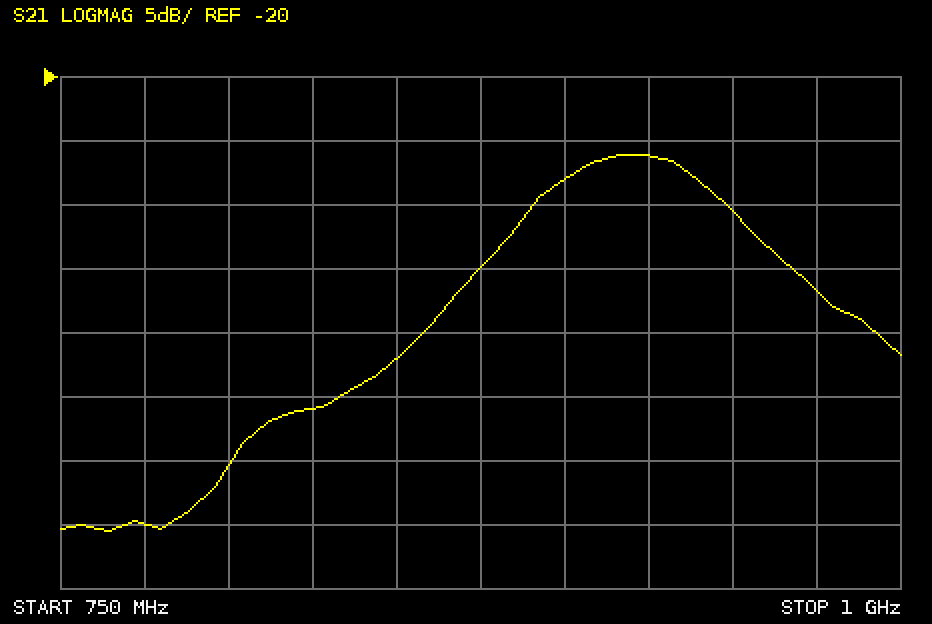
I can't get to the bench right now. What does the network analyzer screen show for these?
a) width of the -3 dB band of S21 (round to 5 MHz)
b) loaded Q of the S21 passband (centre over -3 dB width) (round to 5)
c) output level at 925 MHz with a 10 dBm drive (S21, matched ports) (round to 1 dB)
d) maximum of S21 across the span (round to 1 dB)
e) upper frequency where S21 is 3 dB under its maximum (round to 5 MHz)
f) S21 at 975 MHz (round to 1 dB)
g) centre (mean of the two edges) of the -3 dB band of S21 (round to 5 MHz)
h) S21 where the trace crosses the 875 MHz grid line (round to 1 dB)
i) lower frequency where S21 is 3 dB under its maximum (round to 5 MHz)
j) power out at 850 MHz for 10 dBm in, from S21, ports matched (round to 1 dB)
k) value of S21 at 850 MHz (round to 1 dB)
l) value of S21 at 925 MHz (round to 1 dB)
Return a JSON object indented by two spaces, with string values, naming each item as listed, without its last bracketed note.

{
  "width of the -3 dB band of S21": "50 MHz",
  "loaded Q of the S21 passband (centre over -3 dB width)": "20",
  "output level at 925 MHz with a 10 dBm drive (S21, matched ports)": "-16 dBm",
  "maximum of S21 across the span": "-26 dB",
  "upper frequency where S21 is 3 dB under its maximum": "945 MHz",
  "S21 at 975 MHz": "-37 dB",
  "centre (mean of the two edges) of the -3 dB band of S21": "920 MHz",
  "S21 where the trace crosses the 875 MHz grid line": "-35 dB",
  "lower frequency where S21 is 3 dB under its maximum": "895 MHz",
  "power out at 850 MHz for 10 dBm in, from S21, ports matched": "-32 dBm",
  "value of S21 at 850 MHz": "-42 dB",
  "value of S21 at 925 MHz": "-26 dB"
}
